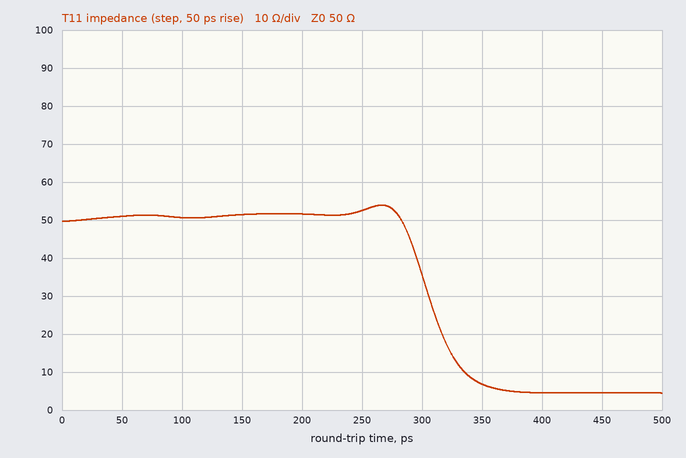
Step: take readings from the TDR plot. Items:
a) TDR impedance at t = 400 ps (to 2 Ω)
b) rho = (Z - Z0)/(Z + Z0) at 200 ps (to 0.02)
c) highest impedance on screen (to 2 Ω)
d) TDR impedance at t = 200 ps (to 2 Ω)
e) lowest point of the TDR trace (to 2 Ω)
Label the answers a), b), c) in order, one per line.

a) 4 Ω
b) +0.02
c) 54 Ω
d) 52 Ω
e) 4 Ω
